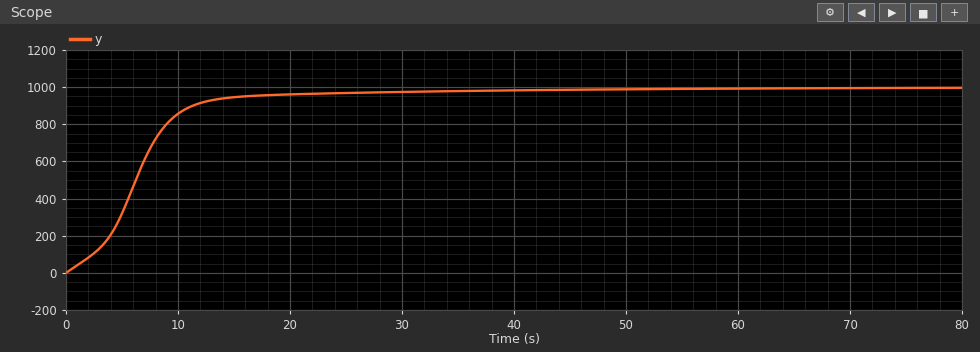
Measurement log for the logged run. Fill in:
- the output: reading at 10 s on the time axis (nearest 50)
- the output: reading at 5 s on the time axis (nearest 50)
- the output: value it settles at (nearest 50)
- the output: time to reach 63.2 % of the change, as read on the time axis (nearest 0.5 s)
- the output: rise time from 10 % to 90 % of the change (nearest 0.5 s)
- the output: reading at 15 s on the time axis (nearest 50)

850
300
1000
7.0 s
9.0 s
950
